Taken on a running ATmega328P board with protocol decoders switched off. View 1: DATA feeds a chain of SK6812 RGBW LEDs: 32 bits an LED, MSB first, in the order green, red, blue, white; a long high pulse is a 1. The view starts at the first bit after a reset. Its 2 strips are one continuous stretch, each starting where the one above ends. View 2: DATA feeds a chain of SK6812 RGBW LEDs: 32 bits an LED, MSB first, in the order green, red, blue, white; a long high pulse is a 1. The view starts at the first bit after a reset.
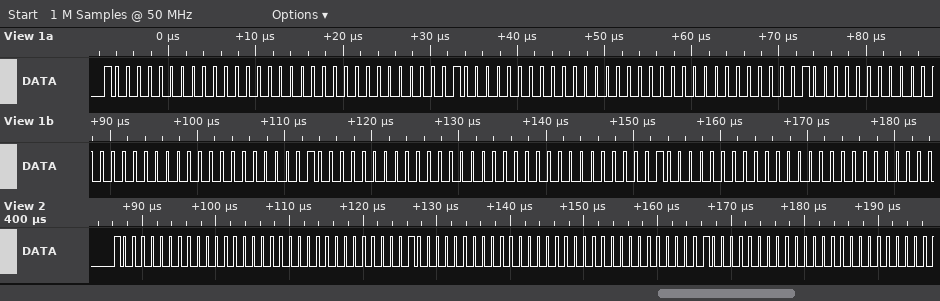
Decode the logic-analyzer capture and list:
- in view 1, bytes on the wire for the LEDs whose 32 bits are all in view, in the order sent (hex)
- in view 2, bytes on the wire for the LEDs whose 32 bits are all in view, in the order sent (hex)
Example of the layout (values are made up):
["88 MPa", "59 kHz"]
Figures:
["80 00 00 00 80 00 00 00 80 00 00 00 80 00 00 00", "80 00 00 00 80 00 00 00"]
